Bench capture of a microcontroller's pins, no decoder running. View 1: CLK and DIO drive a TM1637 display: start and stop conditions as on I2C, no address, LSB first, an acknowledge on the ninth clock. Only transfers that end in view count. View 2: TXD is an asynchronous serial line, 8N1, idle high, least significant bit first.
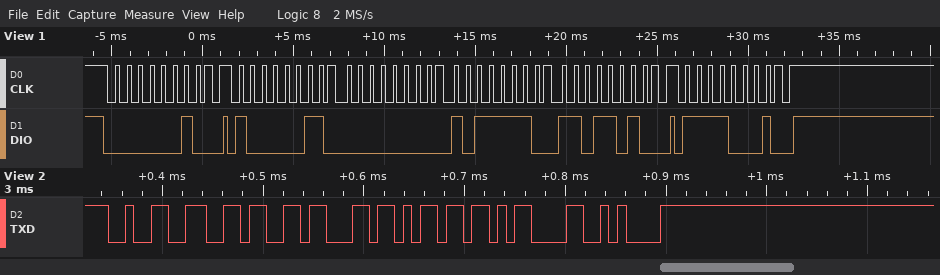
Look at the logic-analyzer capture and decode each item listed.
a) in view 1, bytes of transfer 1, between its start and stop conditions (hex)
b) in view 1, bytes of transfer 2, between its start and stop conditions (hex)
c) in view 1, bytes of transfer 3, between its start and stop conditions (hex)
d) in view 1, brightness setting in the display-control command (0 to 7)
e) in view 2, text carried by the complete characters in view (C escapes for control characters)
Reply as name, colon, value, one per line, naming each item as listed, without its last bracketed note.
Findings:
in view 1, bytes of transfer 1, between its start and stop conditions: 40
in view 1, bytes of transfer 2, between its start and stop conditions: C1 00 7D 5B
in view 1, bytes of transfer 3, between its start and stop conditions: 8F
in view 1, brightness setting in the display-control command: 7
in view 2, text carried by the complete characters in view: "26cm\r\n"
